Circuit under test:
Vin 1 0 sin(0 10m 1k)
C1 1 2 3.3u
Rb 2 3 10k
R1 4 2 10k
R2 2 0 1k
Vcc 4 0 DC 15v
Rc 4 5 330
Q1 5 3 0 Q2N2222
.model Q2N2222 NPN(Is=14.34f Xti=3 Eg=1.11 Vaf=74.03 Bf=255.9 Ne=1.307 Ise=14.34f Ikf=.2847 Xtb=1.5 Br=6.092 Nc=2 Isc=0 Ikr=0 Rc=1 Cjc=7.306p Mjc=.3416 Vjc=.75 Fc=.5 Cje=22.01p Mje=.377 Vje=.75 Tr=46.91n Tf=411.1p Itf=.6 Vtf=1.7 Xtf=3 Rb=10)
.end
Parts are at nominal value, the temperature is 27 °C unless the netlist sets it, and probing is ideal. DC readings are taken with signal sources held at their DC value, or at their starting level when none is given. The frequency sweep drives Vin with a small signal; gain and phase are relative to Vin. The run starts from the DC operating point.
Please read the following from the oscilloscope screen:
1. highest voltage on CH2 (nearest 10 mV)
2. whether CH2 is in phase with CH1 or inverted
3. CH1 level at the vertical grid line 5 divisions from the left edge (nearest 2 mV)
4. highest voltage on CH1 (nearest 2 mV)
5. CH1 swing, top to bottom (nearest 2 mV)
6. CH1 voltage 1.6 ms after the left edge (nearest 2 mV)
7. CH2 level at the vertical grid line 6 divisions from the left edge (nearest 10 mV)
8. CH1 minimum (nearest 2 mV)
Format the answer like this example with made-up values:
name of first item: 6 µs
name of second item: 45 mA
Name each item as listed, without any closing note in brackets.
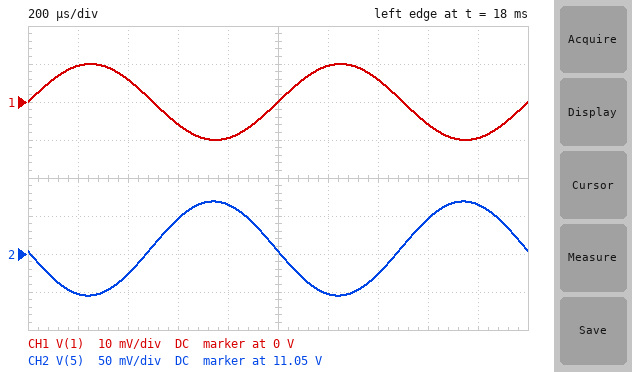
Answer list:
highest voltage on CH2: 11.12 V
whether CH2 is in phase with CH1 or inverted: inverted
CH1 level at the vertical grid line 5 divisions from the left edge: 0 V
highest voltage on CH1: 10 mV
CH1 swing, top to bottom: 20 mV
CH1 voltage 1.6 ms after the left edge: -6 mV
CH2 level at the vertical grid line 6 divisions from the left edge: 11.00 V
CH1 minimum: -10 mV
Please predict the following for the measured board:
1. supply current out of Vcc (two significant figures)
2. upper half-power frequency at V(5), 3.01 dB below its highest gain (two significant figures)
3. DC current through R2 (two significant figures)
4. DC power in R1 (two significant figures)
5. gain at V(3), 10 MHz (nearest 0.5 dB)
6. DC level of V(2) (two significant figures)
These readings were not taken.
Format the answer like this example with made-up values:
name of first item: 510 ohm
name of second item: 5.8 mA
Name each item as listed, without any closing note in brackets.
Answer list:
supply current out of Vcc: 13 mA
upper half-power frequency at V(5), 3.01 dB below its highest gain: 570 kHz
DC current through R2: 1.3 mA
DC power in R1: 19 mW
gain at V(3), 10 MHz: -51.0 dB
DC level of V(2): 1.3 V
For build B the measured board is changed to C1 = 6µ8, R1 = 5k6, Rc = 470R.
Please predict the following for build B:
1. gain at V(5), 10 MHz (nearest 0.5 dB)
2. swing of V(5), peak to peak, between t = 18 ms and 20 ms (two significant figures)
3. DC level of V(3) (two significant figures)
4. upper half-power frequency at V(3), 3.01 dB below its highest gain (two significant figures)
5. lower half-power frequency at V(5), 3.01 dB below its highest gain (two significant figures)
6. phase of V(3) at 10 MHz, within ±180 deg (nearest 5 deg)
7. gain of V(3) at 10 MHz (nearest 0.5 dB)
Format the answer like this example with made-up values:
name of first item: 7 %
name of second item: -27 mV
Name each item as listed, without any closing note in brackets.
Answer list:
gain at V(5), 10 MHz: -11.0 dB
swing of V(5), peak to peak, between t = 18 ms and 20 ms: 140 mV
DC level of V(3): 730 mV
upper half-power frequency at V(3), 3.01 dB below its highest gain: 400 kHz
lower half-power frequency at V(5), 3.01 dB below its highest gain: 30 Hz
phase of V(3) at 10 MHz, within ±180 deg: -35 deg
gain of V(3) at 10 MHz: -57.5 dB
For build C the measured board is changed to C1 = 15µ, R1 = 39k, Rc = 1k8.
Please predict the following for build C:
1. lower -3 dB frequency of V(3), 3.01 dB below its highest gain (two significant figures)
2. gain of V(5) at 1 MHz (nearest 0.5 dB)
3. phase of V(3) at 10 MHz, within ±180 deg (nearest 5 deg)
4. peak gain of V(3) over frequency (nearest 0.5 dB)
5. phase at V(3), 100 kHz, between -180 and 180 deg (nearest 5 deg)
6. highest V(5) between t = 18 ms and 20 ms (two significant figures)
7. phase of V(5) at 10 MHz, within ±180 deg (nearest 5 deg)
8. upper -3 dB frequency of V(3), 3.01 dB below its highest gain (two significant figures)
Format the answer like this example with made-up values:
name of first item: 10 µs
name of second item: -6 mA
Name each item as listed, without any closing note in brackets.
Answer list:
lower -3 dB frequency of V(3), 3.01 dB below its highest gain: 11 Hz
gain of V(5) at 1 MHz: -37.5 dB
phase of V(3) at 10 MHz, within ±180 deg: -85 deg
peak gain of V(3) over frequency: 0 dB
phase at V(3), 100 kHz, between -180 and 180 deg: -10 deg
highest V(5) between t = 18 ms and 20 ms: 15 V
phase of V(5) at 10 MHz, within ±180 deg: -10 deg
upper -3 dB frequency of V(3), 3.01 dB below its highest gain: 510 kHz
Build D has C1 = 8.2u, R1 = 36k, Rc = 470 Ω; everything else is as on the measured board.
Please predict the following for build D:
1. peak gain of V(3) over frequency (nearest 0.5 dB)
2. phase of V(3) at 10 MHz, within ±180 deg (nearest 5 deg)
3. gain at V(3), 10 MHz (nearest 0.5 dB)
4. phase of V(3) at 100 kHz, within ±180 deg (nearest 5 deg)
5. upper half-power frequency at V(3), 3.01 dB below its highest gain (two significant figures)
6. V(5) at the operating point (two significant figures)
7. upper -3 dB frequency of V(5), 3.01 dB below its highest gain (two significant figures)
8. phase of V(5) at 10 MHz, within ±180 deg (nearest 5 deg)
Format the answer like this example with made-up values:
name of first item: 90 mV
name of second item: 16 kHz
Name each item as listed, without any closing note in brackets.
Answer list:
peak gain of V(3) over frequency: 0 dB
phase of V(3) at 10 MHz, within ±180 deg: -85 deg
gain at V(3), 10 MHz: -26.0 dB
phase of V(3) at 100 kHz, within ±180 deg: -10 deg
upper half-power frequency at V(3), 3.01 dB below its highest gain: 500 kHz
V(5) at the operating point: 15 V
upper -3 dB frequency of V(5), 3.01 dB below its highest gain: 140 MHz
phase of V(5) at 10 MHz, within ±180 deg: 0 deg
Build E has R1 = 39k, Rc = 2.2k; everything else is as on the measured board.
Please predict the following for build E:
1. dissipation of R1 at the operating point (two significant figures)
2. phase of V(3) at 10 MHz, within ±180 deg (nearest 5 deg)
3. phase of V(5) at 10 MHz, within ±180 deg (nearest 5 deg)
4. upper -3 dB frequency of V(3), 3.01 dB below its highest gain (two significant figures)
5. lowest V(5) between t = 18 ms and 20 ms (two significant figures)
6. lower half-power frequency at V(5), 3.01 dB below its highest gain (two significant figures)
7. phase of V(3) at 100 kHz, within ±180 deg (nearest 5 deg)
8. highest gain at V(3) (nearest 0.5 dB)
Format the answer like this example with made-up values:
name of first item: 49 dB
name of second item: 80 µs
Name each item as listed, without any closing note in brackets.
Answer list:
dissipation of R1 at the operating point: 5.5 mW
phase of V(3) at 10 MHz, within ±180 deg: -85 deg
phase of V(5) at 10 MHz, within ±180 deg: -15 deg
upper -3 dB frequency of V(3), 3.01 dB below its highest gain: 510 kHz
lowest V(5) between t = 18 ms and 20 ms: 15 V
lower half-power frequency at V(5), 3.01 dB below its highest gain: 480 kHz
phase of V(3) at 100 kHz, within ±180 deg: -10 deg
highest gain at V(3): 0 dB
